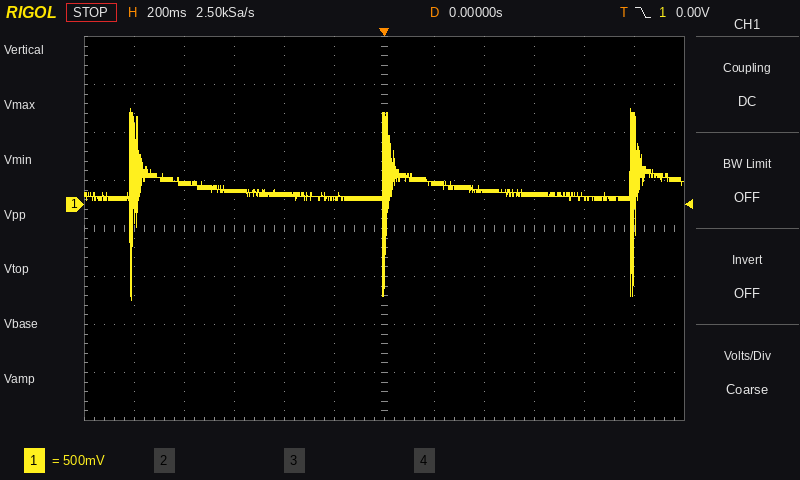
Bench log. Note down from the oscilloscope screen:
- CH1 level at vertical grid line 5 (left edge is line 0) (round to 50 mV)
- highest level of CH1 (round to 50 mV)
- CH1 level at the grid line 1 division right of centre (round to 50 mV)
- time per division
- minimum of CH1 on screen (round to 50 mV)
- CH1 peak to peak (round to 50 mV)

50 mV
1.00 V
200 mV
200 ms
-1.00 V
2.00 V
